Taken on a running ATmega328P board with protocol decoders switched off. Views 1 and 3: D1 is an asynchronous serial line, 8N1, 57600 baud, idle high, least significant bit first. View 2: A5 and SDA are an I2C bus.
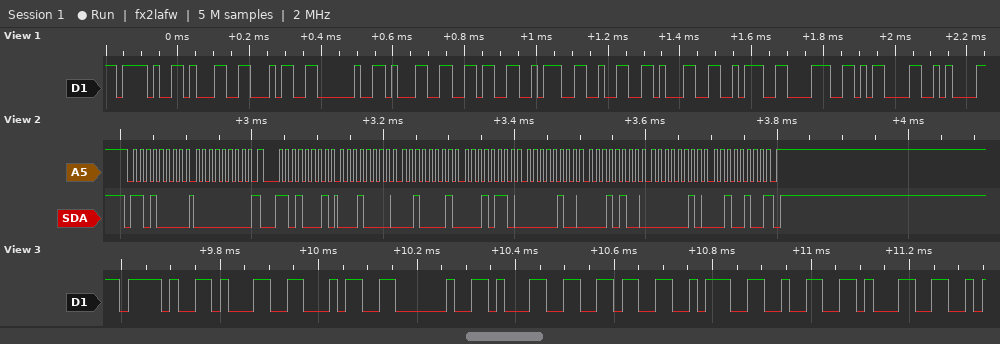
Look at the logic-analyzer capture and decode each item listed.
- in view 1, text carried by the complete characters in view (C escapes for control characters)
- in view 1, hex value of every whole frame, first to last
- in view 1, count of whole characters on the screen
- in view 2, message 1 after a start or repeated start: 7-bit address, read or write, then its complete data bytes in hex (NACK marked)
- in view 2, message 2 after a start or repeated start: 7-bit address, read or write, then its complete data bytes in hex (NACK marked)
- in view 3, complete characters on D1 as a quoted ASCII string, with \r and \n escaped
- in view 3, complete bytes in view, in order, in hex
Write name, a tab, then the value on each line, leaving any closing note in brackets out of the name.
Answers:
in view 1, text carried by the complete characters in view	"/14 16:21:8\r\n"
in view 1, hex value of every whole frame, first to last	2F 31 34 20 31 36 3A 32 31 3A 38 0D 0A
in view 1, count of whole characters on the screen	13
in view 2, message 1 after a start or repeated start: 7-bit address, read or write, then its complete data bytes in hex	0x68 write: 00
in view 2, message 2 after a start or repeated start: 7-bit address, read or write, then its complete data bytes in hex	0x68 read: 10 21 16 04 14 02 24 NACK
in view 3, complete characters on D1 as a quoted ASCII string, with \r and \n escaped	"/14 16:21"
in view 3, complete bytes in view, in order, in hex	0x2F 0x31 0x34 0x20 0x31 0x36 0x3A 0x32 0x31
